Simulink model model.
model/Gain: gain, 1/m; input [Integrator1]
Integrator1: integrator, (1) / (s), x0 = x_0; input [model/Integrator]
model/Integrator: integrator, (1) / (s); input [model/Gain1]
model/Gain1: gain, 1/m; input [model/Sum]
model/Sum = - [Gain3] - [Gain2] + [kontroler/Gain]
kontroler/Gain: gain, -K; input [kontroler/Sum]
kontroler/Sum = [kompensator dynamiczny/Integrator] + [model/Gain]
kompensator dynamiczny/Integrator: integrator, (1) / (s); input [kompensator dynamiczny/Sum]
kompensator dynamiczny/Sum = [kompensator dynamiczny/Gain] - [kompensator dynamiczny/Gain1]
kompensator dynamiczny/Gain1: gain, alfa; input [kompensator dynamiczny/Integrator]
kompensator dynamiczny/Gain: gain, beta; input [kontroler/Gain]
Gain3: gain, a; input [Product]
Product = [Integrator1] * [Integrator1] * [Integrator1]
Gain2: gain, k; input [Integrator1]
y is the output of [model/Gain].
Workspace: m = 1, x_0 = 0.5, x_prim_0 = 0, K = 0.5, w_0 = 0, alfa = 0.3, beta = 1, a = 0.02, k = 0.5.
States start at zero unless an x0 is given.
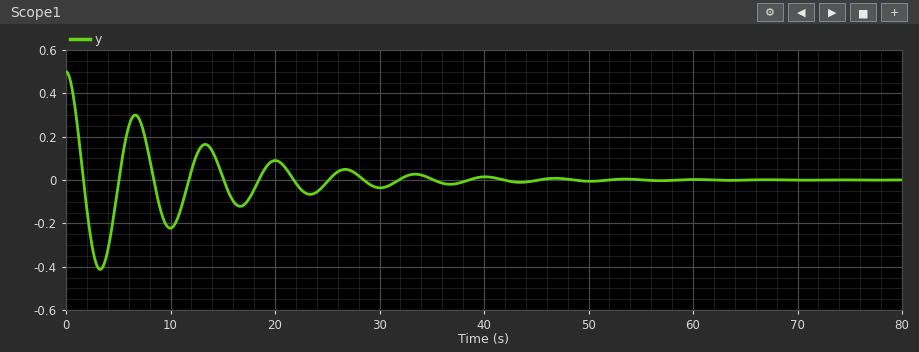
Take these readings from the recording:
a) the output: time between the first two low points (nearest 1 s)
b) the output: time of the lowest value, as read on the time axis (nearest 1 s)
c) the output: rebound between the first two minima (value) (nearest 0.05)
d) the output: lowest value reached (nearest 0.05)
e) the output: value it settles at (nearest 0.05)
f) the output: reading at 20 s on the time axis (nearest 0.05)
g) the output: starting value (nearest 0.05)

7 s
3 s
0.30
-0.40
0.00
0.10
0.50
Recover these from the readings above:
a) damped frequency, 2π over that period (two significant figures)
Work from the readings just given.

0.90 rad/s
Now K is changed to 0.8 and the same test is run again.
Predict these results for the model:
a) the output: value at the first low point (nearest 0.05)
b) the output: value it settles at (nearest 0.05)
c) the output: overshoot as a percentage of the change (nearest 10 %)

-0.35
0.00
70 %
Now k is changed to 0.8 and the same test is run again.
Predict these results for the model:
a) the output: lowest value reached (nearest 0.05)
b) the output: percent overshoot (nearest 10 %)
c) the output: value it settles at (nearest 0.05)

-0.45
90 %
0.00
